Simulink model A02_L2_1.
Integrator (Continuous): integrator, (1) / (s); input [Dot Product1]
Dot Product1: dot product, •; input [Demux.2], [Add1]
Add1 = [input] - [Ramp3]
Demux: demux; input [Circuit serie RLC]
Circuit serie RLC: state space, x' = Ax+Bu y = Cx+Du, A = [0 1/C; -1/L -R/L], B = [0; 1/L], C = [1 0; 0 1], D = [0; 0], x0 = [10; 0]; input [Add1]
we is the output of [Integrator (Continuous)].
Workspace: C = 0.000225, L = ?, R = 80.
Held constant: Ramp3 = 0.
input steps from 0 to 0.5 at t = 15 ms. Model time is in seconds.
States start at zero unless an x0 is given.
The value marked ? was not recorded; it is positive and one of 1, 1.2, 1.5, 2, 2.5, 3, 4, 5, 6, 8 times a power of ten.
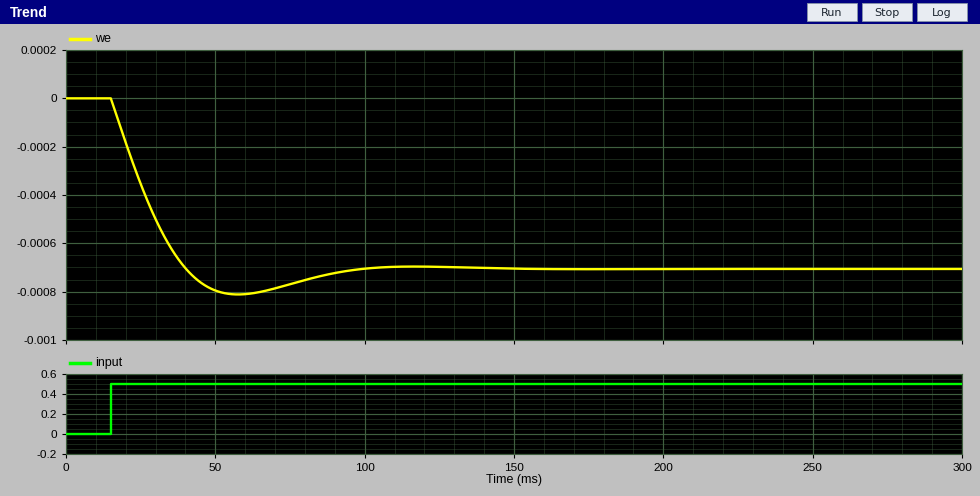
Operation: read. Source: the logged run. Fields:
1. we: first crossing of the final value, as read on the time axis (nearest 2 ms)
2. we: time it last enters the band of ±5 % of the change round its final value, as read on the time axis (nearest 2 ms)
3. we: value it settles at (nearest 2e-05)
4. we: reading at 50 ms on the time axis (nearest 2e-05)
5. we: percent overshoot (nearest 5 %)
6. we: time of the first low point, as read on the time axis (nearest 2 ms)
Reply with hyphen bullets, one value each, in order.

- 40 ms
- 84 ms
- -0.00070
- -0.00080
- 15 %
- 58 ms
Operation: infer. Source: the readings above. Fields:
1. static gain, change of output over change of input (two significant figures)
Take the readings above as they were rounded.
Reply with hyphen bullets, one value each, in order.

- -0.0014
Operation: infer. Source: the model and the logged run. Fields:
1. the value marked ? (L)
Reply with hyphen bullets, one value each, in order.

- 1
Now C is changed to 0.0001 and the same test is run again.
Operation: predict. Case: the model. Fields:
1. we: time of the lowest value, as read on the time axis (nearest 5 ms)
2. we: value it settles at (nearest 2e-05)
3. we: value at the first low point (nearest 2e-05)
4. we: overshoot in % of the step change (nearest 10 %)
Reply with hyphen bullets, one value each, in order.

- 35 ms
- -0.00014
- -0.00028
- 90 %
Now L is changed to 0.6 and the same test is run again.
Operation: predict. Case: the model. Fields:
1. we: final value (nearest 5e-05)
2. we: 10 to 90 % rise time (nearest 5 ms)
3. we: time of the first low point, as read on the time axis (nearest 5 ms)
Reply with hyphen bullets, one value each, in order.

- -0.00060
- 20 ms
- 55 ms
